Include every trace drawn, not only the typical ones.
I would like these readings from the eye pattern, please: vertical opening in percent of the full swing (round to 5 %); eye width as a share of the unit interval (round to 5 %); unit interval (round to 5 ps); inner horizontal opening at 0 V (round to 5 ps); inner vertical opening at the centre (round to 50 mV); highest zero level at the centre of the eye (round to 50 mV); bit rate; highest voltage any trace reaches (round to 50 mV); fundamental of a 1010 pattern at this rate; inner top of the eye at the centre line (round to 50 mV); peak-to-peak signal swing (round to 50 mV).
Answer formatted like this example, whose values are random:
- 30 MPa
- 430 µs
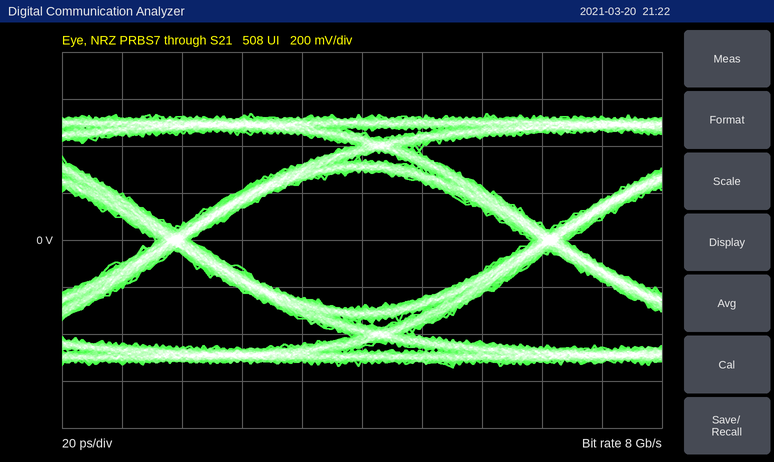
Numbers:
- 55 %
- 90 %
- 125 ps
- 115 ps
- 600 mV
- -300 mV
- 8 Gb/s
- 550 mV
- 4 GHz
- 300 mV
- 1.10 V
